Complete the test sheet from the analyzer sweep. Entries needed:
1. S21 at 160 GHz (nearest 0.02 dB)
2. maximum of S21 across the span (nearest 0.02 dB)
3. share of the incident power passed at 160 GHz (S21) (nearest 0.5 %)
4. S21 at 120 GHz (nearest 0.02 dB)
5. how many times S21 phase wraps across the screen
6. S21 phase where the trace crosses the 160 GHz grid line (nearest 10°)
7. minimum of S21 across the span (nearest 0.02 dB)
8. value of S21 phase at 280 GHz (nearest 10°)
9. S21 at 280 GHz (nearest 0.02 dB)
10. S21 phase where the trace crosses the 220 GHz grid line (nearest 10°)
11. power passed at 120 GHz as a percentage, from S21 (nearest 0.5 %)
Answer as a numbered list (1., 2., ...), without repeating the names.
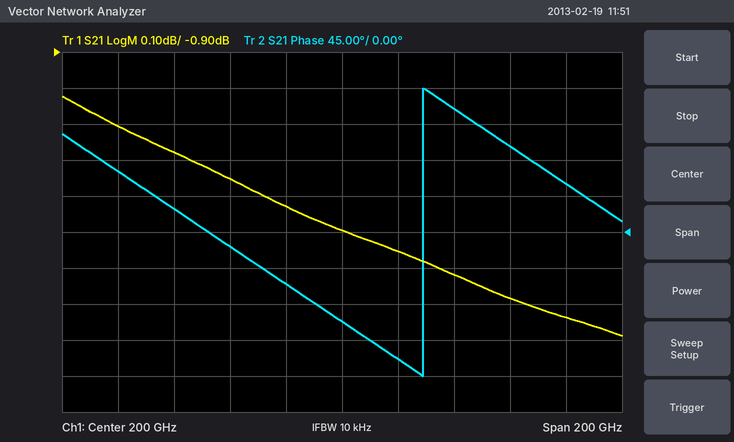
1. -1.26 dB
2. -1.02 dB
3. 75.0 %
4. -1.10 dB
5. 1
6. -20°
7. -1.68 dB
8. 60°
9. -1.64 dB
10. -160°
11. 77.5 %
